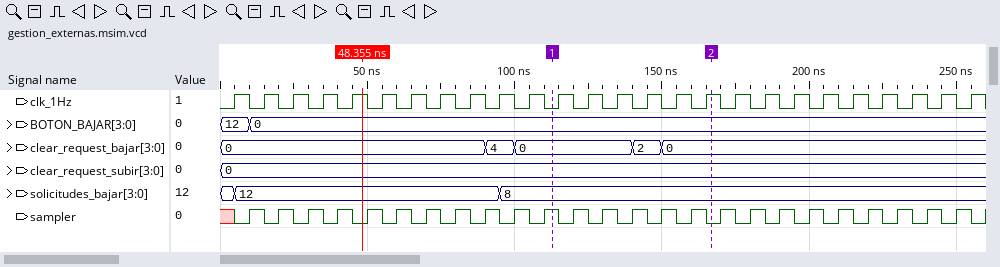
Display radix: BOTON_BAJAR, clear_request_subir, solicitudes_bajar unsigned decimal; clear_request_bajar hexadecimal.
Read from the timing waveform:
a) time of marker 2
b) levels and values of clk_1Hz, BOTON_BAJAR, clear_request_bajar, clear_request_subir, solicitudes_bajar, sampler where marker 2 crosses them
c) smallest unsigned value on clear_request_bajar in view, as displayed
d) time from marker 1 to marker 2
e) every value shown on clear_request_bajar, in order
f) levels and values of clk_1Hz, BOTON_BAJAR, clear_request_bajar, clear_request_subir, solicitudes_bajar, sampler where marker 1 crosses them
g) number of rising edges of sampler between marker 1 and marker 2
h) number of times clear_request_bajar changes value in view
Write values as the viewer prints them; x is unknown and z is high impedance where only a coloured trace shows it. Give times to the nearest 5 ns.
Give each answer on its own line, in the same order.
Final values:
165 ns
clk_1Hz=1, BOTON_BAJAR=0, clear_request_bajar=0, clear_request_subir=0, solicitudes_bajar=8, sampler=0
0
55 ns
0, 4, 0, 2, 0
clk_1Hz=0, BOTON_BAJAR=0, clear_request_bajar=0, clear_request_subir=0, solicitudes_bajar=8, sampler=1
5
4
